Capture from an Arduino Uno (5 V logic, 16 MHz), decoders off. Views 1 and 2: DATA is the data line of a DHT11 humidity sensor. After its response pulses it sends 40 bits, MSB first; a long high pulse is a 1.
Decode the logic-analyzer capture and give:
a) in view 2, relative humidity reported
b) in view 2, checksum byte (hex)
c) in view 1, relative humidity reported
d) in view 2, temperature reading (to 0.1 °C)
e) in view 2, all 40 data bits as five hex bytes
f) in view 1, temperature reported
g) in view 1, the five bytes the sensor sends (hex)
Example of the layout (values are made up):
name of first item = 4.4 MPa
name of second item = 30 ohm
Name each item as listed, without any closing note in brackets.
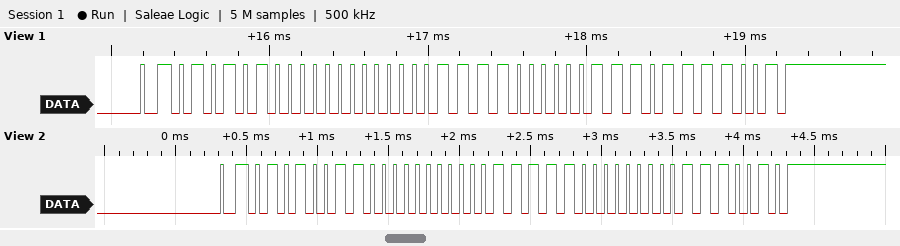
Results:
in view 2, relative humidity reported = 83 %
in view 2, checksum byte = 0x72
in view 1, relative humidity reported = 84 %
in view 2, temperature reading = 31.0 °C
in view 2, all 40 data bits as five hex bytes = 53 00 1F 00 72
in view 1, temperature reported = 30.7 °C
in view 1, the five bytes the sensor sends = 54 00 1E 07 79
